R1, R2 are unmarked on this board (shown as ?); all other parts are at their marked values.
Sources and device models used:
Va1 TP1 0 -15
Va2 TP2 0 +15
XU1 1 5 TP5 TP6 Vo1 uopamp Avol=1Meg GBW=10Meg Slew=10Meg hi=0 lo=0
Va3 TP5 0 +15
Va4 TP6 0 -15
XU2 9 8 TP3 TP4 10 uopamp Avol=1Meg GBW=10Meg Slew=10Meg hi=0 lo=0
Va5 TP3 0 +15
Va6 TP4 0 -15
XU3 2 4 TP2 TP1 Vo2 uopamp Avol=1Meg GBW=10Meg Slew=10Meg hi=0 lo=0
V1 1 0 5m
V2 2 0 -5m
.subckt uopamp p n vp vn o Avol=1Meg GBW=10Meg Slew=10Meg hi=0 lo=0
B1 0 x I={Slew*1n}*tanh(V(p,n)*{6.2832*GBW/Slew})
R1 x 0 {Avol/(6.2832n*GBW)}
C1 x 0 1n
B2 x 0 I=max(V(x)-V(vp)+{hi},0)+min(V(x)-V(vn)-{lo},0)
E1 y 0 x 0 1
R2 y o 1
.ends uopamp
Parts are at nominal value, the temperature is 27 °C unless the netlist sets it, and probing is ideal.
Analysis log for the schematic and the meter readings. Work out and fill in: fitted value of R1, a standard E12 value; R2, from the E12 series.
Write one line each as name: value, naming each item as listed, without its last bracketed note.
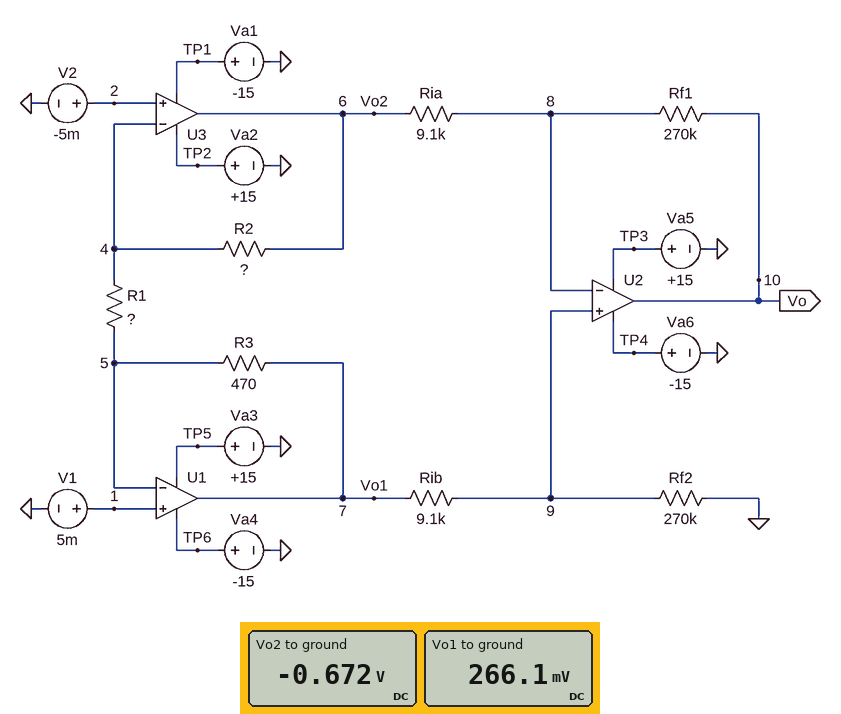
fitted value of R1, a standard E12 value: 18 Ω
R2, from the E12 series: 1.2 kΩ
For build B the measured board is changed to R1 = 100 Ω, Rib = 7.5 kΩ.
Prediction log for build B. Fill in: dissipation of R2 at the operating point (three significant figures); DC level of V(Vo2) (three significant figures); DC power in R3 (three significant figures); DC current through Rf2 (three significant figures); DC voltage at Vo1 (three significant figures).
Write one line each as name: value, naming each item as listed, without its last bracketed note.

dissipation of R2 at the operating point: 12.0 µW
DC level of V(Vo2): -125 mV
DC power in R3: 4.70 µW
DC current through Rf2: 187 nA
DC voltage at Vo1: 52.0 mV
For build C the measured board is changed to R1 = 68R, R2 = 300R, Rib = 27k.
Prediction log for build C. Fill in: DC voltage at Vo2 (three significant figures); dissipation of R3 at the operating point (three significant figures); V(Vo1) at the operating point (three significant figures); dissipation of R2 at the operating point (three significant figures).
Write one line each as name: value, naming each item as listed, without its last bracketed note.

DC voltage at Vo2: -49.1 mV
dissipation of R3 at the operating point: 10.2 µW
V(Vo1) at the operating point: 74.1 mV
dissipation of R2 at the operating point: 6.49 µW
